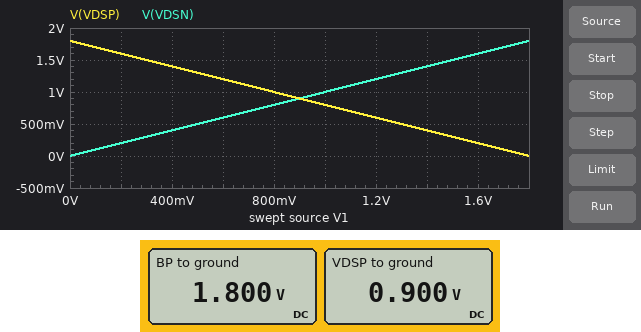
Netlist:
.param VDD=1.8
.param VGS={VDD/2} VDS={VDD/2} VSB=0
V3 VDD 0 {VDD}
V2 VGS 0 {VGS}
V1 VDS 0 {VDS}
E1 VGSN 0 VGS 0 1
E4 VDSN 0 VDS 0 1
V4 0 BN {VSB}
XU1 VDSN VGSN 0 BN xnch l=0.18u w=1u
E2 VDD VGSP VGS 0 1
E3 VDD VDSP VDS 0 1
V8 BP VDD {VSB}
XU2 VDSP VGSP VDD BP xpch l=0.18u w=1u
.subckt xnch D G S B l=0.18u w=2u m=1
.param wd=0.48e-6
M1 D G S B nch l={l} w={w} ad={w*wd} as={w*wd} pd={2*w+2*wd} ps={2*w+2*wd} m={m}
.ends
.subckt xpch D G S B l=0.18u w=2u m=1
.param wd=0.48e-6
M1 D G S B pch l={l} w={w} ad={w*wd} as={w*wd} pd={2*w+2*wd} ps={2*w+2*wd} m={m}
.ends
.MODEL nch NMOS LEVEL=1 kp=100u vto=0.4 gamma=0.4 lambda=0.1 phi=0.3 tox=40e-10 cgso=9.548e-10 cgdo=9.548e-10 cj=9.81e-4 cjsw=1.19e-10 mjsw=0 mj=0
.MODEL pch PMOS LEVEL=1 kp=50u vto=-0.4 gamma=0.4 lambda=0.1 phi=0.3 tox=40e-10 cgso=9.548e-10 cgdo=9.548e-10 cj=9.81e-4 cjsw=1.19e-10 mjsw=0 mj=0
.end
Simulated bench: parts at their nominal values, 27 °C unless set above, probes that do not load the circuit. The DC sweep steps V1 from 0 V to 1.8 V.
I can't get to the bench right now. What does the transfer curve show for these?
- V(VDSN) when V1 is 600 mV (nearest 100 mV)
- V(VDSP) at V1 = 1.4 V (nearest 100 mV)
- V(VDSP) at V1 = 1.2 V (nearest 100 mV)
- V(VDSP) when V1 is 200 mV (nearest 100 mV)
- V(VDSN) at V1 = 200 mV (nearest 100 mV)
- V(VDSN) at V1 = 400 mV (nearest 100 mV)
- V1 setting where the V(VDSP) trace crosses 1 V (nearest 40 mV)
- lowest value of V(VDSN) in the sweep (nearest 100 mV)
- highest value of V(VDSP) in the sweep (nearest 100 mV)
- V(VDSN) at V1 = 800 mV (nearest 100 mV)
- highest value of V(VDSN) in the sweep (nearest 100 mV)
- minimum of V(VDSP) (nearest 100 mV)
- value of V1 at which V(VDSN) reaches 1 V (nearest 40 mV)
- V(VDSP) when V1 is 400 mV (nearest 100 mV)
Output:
600 mV
400 mV
600 mV
1.6 V
200 mV
400 mV
800 mV
0 V
1.8 V
800 mV
1.8 V
0 V
1.00 V
1.4 V
